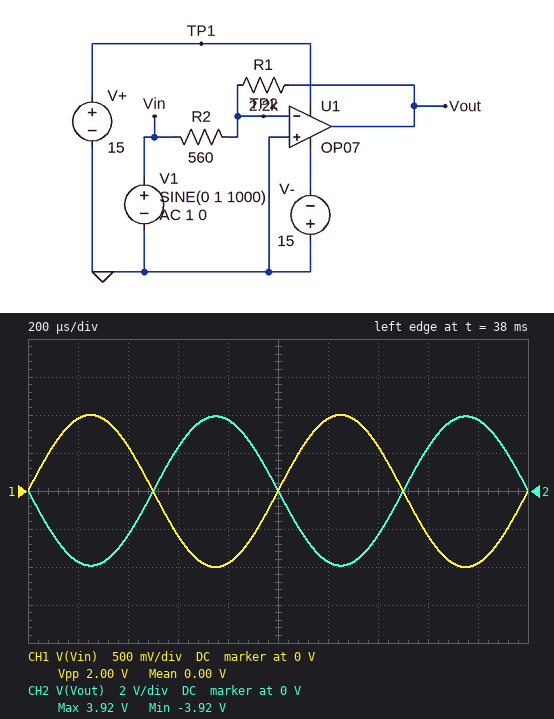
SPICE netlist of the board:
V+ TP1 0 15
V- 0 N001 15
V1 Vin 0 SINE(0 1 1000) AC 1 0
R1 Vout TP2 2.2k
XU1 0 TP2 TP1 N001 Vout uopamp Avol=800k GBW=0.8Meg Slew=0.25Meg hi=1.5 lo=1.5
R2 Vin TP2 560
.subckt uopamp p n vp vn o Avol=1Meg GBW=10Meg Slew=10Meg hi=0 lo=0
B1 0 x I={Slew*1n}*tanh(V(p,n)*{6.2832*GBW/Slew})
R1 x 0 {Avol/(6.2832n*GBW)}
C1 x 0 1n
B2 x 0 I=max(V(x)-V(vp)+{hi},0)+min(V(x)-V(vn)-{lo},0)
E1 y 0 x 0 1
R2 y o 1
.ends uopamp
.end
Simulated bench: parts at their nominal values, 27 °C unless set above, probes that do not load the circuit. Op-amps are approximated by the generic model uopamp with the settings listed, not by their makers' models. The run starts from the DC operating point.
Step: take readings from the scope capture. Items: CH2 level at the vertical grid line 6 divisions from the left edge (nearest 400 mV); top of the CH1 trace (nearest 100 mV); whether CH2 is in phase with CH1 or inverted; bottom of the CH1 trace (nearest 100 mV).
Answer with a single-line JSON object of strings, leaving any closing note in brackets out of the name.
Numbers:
{"CH2 level at the vertical grid line 6 divisions from the left edge": "-3.6 V", "top of the CH1 trace": "1.0 V", "whether CH2 is in phase with CH1 or inverted": "inverted", "bottom of the CH1 trace": "-1.0 V"}
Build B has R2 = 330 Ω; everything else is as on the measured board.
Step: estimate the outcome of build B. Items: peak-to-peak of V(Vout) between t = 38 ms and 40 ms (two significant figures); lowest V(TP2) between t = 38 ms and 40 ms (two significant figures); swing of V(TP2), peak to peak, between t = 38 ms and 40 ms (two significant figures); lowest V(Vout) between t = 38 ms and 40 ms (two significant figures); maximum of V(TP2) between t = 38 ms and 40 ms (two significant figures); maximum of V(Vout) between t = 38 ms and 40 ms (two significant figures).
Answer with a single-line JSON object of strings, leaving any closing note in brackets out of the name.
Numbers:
{"peak-to-peak of V(Vout) between t = 38 ms and 40 ms": "13 V", "lowest V(TP2) between t = 38 ms and 40 ms": "-8.4 mV", "swing of V(TP2), peak to peak, between t = 38 ms and 40 ms": "17 mV", "lowest V(Vout) between t = 38 ms and 40 ms": "-6.7 V", "maximum of V(TP2) between t = 38 ms and 40 ms": "8.4 mV", "maximum of V(Vout) between t = 38 ms and 40 ms": "6.7 V"}
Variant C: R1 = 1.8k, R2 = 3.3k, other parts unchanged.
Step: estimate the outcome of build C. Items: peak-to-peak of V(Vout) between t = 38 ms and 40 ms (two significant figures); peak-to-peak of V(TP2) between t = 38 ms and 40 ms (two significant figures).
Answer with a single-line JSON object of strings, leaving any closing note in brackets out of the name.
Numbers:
{"peak-to-peak of V(Vout) between t = 38 ms and 40 ms": "1.1 V", "peak-to-peak of V(TP2) between t = 38 ms and 40 ms": "1.4 mV"}
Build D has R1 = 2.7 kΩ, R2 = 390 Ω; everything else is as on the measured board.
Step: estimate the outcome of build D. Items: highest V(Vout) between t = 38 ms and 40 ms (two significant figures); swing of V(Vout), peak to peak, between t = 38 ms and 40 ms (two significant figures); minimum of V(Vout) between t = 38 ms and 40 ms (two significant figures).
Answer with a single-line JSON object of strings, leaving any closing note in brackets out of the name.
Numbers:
{"highest V(Vout) between t = 38 ms and 40 ms": "6.9 V", "swing of V(Vout), peak to peak, between t = 38 ms and 40 ms": "14 V", "minimum of V(Vout) between t = 38 ms and 40 ms": "-6.9 V"}
